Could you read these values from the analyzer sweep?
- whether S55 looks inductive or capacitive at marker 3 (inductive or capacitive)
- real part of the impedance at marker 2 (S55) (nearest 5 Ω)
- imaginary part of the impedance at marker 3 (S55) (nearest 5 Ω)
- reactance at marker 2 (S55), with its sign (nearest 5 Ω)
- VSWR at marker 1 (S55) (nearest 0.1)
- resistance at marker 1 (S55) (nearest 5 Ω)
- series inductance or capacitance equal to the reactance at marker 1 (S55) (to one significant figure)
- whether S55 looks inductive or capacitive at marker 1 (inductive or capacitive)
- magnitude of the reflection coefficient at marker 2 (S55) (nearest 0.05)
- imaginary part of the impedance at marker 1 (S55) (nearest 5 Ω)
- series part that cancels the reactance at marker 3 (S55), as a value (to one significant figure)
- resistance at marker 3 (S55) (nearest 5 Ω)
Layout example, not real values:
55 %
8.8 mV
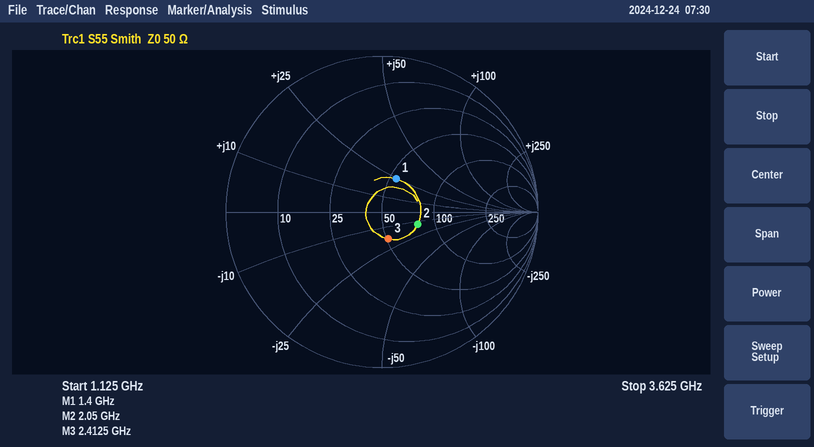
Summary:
capacitive
80 Ω
-20 Ω
-15 Ω
1.6
55 Ω
3 nH
inductive
0.25
+25 Ω
1 nH
50 Ω
